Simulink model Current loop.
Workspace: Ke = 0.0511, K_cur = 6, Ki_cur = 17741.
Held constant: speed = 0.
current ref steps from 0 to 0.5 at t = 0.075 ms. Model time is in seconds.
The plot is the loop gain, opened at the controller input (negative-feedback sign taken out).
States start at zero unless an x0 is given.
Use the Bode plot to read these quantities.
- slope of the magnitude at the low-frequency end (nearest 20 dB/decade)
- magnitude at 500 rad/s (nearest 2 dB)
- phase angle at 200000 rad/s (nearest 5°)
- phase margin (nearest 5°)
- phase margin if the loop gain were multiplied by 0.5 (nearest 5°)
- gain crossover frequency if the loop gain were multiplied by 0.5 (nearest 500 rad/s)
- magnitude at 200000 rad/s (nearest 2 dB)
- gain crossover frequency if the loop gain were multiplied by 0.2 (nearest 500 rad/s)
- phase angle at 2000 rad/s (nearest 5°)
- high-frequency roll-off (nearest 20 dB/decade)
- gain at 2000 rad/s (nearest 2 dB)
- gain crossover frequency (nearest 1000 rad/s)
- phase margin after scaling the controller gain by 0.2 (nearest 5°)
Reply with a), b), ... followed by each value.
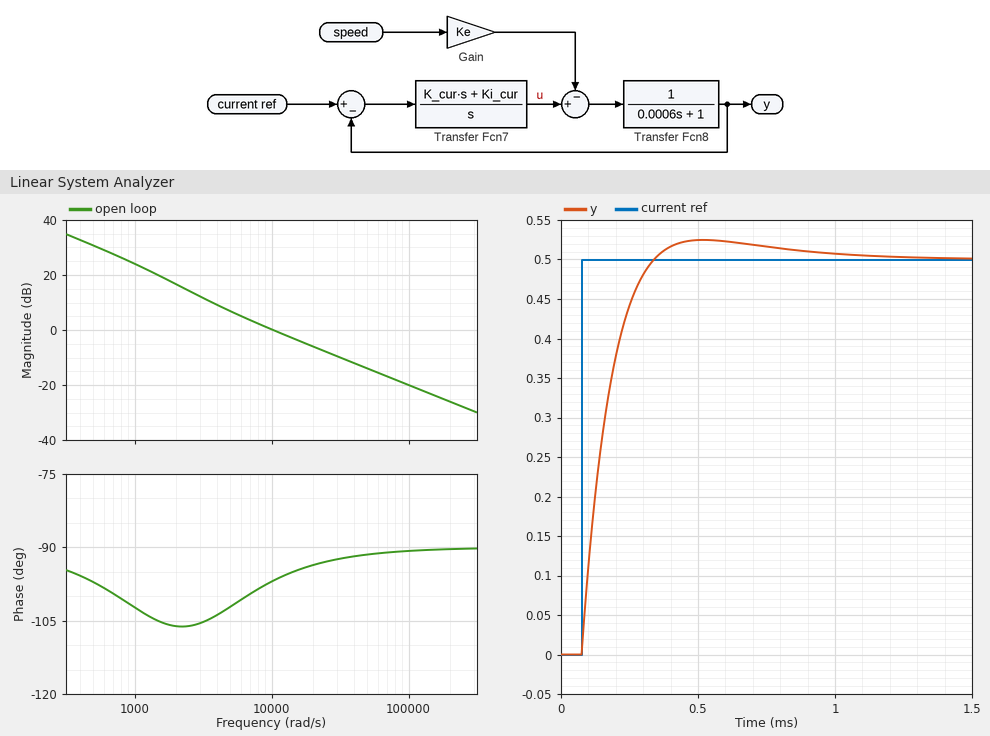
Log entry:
a) -20 dB/decade
b) 30 dB
c) -90°
d) 85°
e) 80°
f) 5500 rad/s
g) -26 dB
h) 2500 rad/s
i) -105°
j) -20 dB/decade
k) 16 dB
l) 10000 rad/s
m) 75°
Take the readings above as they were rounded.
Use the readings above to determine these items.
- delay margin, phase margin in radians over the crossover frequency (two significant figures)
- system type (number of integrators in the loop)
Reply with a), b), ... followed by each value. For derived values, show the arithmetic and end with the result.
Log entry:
a) 85 × π / 180 / 10000 = 0.00015 s
b) 1
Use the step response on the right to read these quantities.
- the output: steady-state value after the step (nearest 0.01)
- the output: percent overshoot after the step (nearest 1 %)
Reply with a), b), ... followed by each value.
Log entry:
a) 0.50
b) 5 %
